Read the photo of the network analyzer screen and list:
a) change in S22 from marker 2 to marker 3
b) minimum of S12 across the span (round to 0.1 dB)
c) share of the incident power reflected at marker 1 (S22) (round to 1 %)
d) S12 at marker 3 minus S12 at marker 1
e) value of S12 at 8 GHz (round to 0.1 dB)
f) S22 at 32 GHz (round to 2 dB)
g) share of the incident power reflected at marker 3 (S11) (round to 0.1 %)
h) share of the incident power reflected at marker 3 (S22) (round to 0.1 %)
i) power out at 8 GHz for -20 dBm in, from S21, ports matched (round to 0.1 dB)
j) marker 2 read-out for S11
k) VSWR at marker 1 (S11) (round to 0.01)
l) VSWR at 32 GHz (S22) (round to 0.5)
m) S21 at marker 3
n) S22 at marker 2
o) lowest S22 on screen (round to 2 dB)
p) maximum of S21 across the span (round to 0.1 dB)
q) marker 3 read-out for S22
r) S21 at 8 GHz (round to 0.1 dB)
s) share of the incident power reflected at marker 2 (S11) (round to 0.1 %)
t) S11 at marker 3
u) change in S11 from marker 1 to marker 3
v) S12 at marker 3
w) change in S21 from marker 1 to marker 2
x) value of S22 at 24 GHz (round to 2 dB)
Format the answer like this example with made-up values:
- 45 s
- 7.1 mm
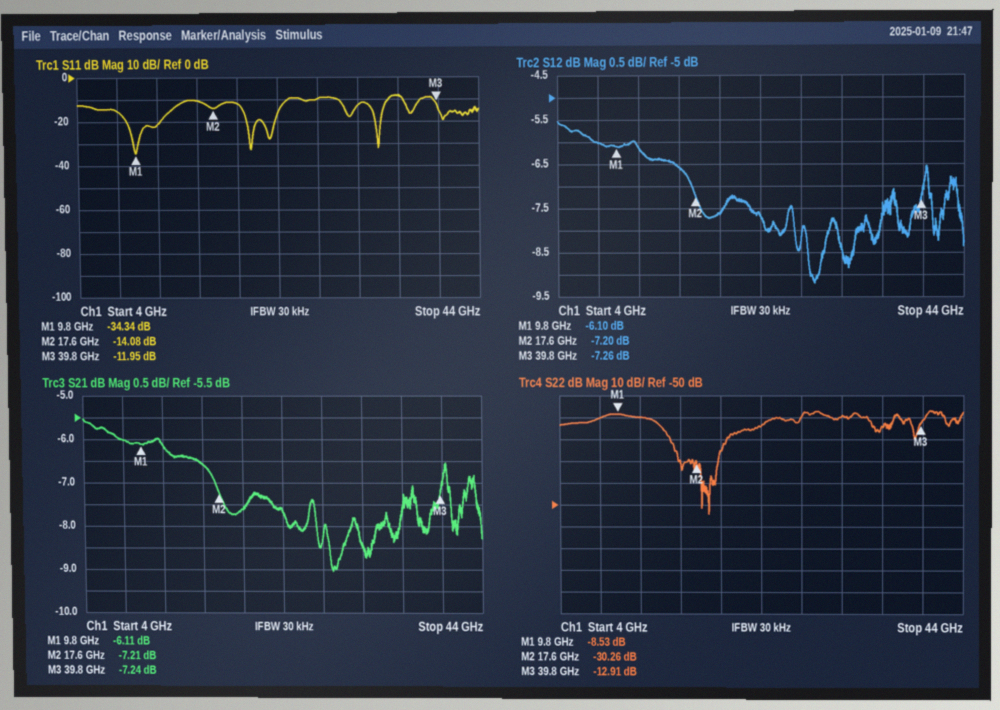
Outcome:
- 17.35 dB
- -9.2 dB
- 14 %
- -1.16 dB
- -6.0 dB
- -10 dB
- 6.4 %
- 5.1 %
- -26.0 dBm
- -14.08 dB
- 1.04
- 2.0
- -7.24 dB
- -30.26 dB
- -54 dB
- -5.5 dB
- -12.91 dB
- -6.0 dB
- 3.9 %
- -11.95 dB
- 22.39 dB
- -7.26 dB
- -1.10 dB
- -14 dB
